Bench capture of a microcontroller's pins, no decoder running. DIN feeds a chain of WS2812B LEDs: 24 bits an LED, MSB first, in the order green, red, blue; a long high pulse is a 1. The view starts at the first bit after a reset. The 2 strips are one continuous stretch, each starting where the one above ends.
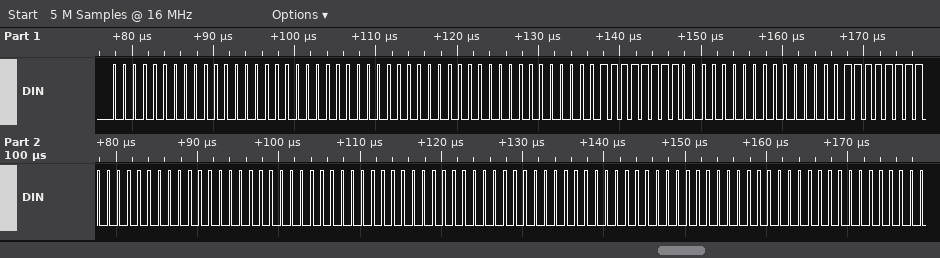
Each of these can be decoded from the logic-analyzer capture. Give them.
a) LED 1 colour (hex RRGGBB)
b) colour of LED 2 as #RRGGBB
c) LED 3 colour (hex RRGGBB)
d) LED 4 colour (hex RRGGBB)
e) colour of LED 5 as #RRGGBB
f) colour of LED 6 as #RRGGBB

#000000
#000000
#00FF00
#00FF00
#000000
#000000
